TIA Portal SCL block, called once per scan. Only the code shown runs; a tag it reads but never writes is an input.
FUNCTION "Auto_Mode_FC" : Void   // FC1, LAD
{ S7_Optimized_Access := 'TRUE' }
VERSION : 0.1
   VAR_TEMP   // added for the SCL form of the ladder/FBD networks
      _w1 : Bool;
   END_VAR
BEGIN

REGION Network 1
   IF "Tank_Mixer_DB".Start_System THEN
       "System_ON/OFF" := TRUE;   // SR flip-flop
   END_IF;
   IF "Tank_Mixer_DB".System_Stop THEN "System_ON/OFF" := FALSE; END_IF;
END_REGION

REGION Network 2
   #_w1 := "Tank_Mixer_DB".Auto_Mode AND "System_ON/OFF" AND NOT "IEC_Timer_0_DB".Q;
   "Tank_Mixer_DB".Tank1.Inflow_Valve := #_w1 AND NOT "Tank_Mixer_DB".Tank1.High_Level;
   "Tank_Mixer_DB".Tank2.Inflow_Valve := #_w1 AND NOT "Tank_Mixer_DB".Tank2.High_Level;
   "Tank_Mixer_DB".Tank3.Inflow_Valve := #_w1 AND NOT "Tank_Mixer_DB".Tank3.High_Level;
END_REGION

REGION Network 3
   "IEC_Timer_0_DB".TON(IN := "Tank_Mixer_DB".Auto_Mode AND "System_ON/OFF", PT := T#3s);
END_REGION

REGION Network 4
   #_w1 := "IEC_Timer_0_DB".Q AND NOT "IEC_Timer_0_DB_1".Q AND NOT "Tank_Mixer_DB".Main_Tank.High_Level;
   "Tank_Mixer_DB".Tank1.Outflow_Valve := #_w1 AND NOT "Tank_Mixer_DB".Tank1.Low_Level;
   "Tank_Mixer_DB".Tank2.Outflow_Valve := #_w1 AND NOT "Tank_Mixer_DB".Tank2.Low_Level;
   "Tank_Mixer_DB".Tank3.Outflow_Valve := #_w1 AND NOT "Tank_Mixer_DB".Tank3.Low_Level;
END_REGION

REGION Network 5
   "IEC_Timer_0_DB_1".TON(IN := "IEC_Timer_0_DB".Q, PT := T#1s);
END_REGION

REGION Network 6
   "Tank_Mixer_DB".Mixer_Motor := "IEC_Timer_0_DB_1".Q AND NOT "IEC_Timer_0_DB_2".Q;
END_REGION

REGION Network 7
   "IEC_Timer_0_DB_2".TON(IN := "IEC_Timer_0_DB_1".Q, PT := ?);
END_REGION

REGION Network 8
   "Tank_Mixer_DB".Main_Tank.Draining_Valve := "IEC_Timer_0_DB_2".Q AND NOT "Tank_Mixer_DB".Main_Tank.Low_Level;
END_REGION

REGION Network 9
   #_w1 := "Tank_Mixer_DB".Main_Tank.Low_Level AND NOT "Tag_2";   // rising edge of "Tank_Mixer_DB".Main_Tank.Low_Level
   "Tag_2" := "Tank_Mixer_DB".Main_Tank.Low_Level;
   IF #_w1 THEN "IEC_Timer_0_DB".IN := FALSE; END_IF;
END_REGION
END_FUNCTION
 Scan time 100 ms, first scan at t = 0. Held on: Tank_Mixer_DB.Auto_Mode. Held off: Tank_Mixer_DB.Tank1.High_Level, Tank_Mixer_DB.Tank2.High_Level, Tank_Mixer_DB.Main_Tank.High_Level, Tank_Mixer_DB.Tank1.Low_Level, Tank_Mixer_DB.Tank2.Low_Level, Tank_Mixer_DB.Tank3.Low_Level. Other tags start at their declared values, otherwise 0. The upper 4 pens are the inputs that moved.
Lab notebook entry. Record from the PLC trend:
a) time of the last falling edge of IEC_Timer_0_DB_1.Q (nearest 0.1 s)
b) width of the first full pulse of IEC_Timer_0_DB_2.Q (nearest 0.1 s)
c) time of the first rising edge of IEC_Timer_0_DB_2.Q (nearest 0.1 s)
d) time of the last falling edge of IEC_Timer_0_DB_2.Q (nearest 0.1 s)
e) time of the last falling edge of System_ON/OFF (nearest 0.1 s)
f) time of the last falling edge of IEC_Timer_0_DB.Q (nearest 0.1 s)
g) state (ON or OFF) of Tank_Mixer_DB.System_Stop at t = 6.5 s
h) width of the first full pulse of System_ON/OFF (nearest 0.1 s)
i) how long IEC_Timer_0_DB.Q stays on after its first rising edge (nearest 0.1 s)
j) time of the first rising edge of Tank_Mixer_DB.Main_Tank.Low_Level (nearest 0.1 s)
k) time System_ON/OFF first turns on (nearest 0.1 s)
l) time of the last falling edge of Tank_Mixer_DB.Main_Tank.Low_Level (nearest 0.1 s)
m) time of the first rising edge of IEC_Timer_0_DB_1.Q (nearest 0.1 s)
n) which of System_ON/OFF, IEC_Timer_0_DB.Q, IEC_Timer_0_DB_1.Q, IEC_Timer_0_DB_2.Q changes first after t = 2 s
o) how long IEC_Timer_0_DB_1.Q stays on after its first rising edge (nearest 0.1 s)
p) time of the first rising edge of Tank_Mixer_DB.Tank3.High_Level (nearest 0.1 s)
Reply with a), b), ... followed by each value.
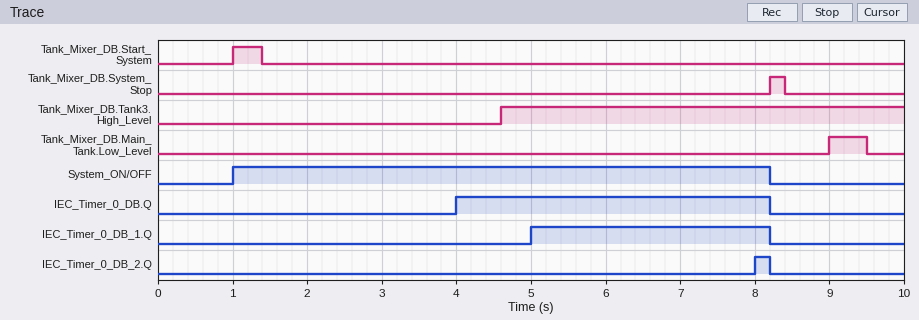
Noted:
a) 8.2 s
b) 0.2 s
c) 8.0 s
d) 8.2 s
e) 8.2 s
f) 8.2 s
g) OFF
h) 7.2 s
i) 4.2 s
j) 9.0 s
k) 1.0 s
l) 9.5 s
m) 5.0 s
n) IEC_Timer_0_DB.Q
o) 3.2 s
p) 4.6 s
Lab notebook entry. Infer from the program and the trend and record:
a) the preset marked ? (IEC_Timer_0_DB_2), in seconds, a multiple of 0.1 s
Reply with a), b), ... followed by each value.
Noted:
a) 3.0 s
